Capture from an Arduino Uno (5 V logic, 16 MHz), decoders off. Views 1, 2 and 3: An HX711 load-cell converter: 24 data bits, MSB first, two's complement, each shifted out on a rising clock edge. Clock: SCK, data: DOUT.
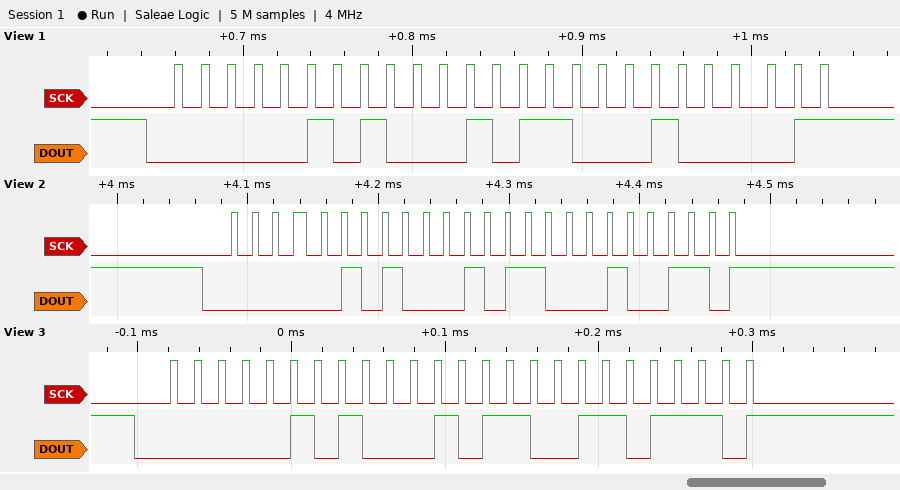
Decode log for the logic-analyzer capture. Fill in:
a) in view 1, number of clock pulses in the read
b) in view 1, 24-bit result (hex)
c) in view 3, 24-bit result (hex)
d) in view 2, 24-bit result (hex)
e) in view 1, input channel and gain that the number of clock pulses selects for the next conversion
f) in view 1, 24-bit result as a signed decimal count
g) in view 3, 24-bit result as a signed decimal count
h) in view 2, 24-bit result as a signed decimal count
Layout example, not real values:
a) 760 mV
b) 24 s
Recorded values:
a) 25
b) 0x051621
c) 0x05166E
d) 0x051626
e) channel A, gain 128
f) 333345
g) 333422
h) 333350
